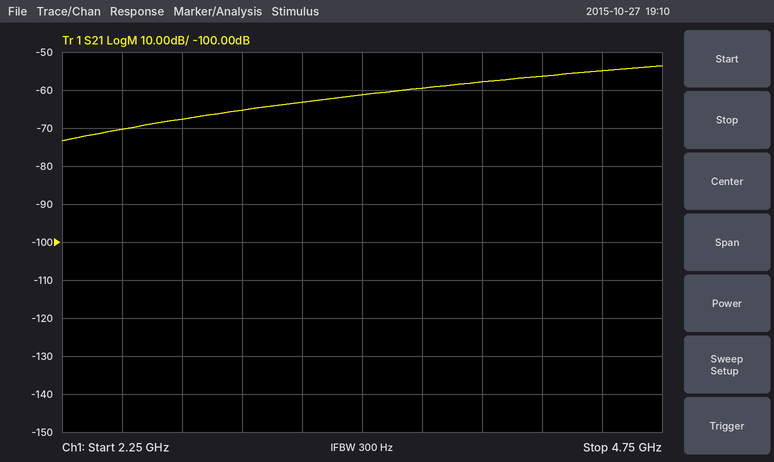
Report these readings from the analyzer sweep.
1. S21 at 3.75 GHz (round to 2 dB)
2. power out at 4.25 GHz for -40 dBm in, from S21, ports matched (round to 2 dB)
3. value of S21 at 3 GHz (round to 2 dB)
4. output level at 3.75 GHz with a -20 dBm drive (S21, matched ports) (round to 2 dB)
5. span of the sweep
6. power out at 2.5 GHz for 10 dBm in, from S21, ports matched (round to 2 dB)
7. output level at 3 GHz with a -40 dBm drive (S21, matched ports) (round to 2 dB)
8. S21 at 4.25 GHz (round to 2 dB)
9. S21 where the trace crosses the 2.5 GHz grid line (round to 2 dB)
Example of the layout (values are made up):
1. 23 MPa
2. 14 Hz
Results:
1. -60 dB
2. -96 dBm
3. -66 dB
4. -80 dBm
5. 2.5 GHz
6. -60 dBm
7. -106 dBm
8. -56 dB
9. -70 dB
